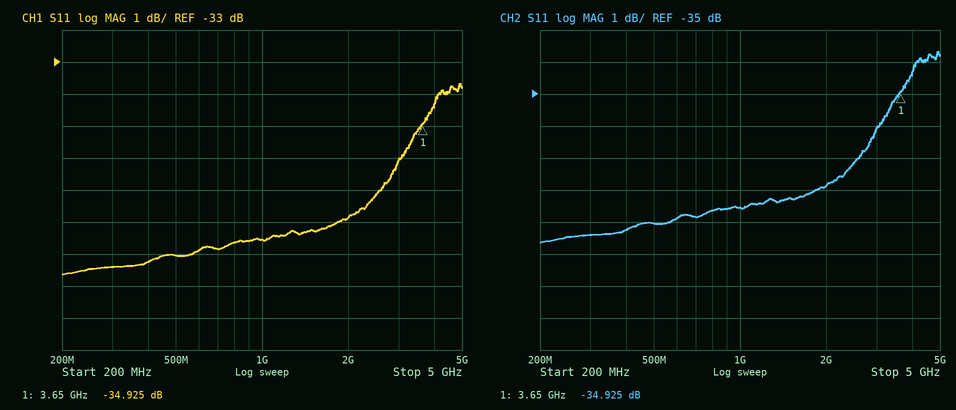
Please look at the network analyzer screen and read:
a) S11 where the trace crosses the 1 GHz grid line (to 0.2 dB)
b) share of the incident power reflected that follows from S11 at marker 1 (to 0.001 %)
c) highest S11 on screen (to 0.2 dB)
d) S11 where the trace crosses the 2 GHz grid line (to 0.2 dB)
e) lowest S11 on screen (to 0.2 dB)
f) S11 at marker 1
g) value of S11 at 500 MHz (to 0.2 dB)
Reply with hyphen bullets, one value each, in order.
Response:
- -38.6 dB
- 0.032 %
- -33.6 dB
- -37.8 dB
- -39.6 dB
- -34.925 dB
- -39.0 dB
